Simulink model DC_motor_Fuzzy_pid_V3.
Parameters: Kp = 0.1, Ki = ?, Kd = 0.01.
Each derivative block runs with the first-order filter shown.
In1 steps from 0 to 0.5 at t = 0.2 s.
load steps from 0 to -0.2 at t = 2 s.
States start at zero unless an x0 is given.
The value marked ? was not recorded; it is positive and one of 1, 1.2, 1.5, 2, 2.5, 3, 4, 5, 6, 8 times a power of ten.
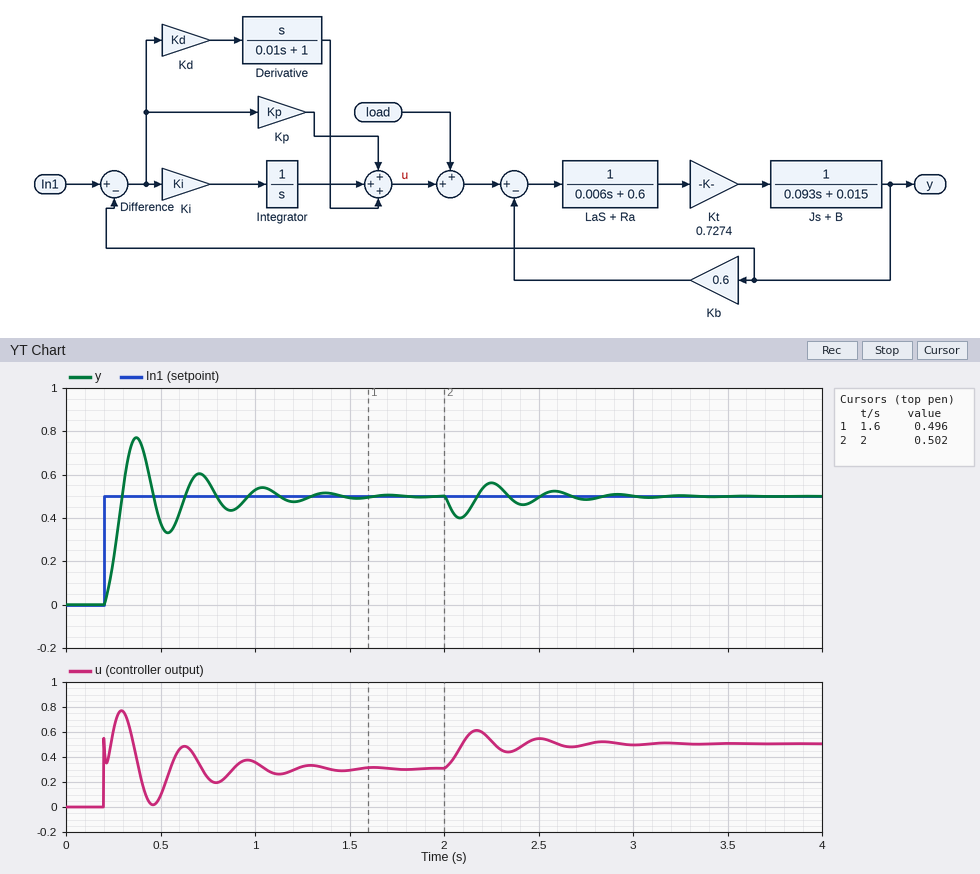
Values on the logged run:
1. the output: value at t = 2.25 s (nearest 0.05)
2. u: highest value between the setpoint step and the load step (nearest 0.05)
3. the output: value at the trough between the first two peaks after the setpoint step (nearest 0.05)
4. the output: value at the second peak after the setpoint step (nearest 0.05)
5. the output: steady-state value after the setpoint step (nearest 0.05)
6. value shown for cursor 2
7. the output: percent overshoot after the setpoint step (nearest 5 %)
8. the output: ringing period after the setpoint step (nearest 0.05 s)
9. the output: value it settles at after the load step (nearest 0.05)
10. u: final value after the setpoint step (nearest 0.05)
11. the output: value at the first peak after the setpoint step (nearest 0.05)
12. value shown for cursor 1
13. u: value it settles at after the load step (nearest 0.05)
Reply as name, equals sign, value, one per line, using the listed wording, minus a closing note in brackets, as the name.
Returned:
the output: value at t = 2.25 s = 0.55
u: highest value between the setpoint step and the load step = 0.75
the output: value at the trough between the first two peaks after the setpoint step = 0.35
the output: value at the second peak after the setpoint step = 0.60
the output: steady-state value after the setpoint step = 0.50
value shown for cursor 2 = 0.502
the output: percent overshoot after the setpoint step = 55 %
the output: ringing period after the setpoint step = 0.35 s
the output: value it settles at after the load step = 0.50
u: final value after the setpoint step = 0.30
the output: value at the first peak after the setpoint step = 0.75
value shown for cursor 1 = 0.496
u: value it settles at after the load step = 0.50
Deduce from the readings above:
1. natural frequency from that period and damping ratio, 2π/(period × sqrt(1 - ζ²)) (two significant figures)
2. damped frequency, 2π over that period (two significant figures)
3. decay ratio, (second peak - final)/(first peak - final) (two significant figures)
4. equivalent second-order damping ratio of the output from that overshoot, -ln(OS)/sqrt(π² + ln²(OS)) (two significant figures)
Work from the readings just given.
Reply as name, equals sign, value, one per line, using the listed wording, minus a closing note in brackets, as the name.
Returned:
natural frequency from that period and damping ratio, 2π/(period × sqrt(1 - ζ²)) = 18 rad/s
damped frequency, 2π over that period = 18 rad/s
decay ratio, (second peak - final)/(first peak - final) = 0.40
equivalent second-order damping ratio of the output from that overshoot, -ln(OS)/sqrt(π² + ln²(OS)) = 0.19
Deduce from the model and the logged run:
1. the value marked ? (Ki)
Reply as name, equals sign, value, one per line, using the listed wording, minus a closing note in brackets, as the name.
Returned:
the value marked ? = 30
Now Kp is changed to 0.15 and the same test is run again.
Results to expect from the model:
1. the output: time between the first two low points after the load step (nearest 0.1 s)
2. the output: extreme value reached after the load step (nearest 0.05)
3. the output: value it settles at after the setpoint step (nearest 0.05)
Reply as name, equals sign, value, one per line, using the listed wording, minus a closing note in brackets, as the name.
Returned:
the output: time between the first two low points after the load step = 0.3 s
the output: extreme value reached after the load step = 0.40
the output: value it settles at after the setpoint step = 0.50
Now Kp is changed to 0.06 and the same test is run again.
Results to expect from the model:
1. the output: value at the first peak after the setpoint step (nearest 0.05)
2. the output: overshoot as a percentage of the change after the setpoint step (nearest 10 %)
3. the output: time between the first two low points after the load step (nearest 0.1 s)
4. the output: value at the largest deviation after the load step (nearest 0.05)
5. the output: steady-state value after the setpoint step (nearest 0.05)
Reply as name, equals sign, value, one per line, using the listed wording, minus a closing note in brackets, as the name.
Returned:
the output: value at the first peak after the setpoint step = 0.80
the output: overshoot as a percentage of the change after the setpoint step = 60 %
the output: time between the first two low points after the load step = 0.3 s
the output: value at the largest deviation after the load step = 0.40
the output: steady-state value after the setpoint step = 0.50
